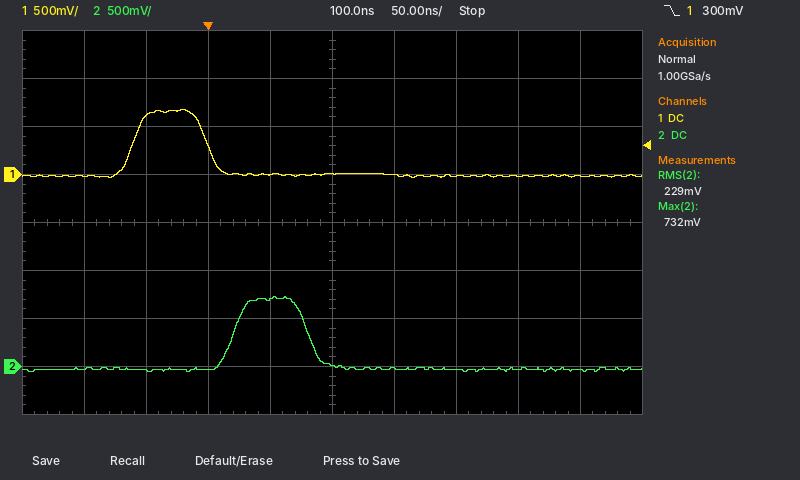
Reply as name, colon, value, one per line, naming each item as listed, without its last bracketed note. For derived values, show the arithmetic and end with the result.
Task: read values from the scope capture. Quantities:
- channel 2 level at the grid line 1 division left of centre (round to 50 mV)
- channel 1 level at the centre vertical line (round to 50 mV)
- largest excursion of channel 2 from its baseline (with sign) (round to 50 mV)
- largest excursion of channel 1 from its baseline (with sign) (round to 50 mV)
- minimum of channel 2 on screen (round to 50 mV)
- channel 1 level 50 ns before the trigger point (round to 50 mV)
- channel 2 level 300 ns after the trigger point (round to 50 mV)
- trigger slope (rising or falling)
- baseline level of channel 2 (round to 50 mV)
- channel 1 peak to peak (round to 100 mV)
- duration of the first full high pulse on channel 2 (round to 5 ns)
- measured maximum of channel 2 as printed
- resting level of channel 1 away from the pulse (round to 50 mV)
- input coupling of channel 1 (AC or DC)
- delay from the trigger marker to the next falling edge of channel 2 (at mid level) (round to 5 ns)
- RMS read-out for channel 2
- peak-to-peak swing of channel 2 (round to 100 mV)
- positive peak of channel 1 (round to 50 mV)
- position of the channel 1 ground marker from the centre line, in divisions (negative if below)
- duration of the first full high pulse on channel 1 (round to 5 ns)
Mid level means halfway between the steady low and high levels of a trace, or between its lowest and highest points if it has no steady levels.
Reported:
channel 2 level at the grid line 1 division left of centre: 700 mV
channel 1 level at the centre vertical line: 0 mV
largest excursion of channel 2 from its baseline (with sign): +750 mV
largest excursion of channel 1 from its baseline (with sign): 700 mV − (0 mV) = +700 mV
minimum of channel 2 on screen: -50 mV
channel 1 level 50 ns before the trigger point: 600 mV
channel 2 level 300 ns after the trigger point: -50 mV
trigger slope: falling
baseline level of channel 2: -50 mV
channel 1 peak to peak: 700 mV
duration of the first full high pulse on channel 2: 60 ns
measured maximum of channel 2 as printed: 732 mV
resting level of channel 1 away from the pulse: 0 mV
input coupling of channel 1: DC
delay from the trigger marker to the next falling edge of channel 2 (at mid level): 80 ns
RMS read-out for channel 2: 229 mV
peak-to-peak swing of channel 2: 800 mV
positive peak of channel 1: 700 mV
position of the channel 1 ground marker from the centre line, in divisions: +1.0 div
duration of the first full high pulse on channel 1: 60 ns
